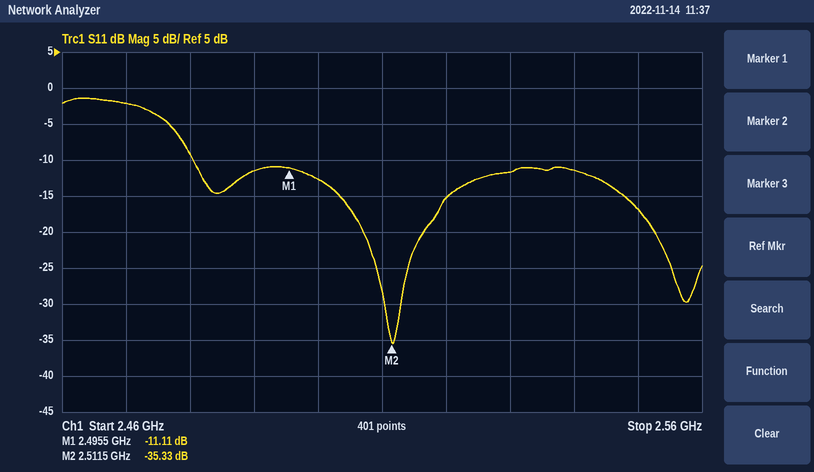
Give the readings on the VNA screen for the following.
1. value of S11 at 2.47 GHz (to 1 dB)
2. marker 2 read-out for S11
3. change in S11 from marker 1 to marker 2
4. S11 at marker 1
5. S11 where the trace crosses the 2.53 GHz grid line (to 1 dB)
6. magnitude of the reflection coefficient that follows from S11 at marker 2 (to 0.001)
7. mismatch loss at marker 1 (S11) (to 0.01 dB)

-2 dB
-35.33 dB
-24.22 dB
-11.11 dB
-12 dB
0.017
0.35 dB
